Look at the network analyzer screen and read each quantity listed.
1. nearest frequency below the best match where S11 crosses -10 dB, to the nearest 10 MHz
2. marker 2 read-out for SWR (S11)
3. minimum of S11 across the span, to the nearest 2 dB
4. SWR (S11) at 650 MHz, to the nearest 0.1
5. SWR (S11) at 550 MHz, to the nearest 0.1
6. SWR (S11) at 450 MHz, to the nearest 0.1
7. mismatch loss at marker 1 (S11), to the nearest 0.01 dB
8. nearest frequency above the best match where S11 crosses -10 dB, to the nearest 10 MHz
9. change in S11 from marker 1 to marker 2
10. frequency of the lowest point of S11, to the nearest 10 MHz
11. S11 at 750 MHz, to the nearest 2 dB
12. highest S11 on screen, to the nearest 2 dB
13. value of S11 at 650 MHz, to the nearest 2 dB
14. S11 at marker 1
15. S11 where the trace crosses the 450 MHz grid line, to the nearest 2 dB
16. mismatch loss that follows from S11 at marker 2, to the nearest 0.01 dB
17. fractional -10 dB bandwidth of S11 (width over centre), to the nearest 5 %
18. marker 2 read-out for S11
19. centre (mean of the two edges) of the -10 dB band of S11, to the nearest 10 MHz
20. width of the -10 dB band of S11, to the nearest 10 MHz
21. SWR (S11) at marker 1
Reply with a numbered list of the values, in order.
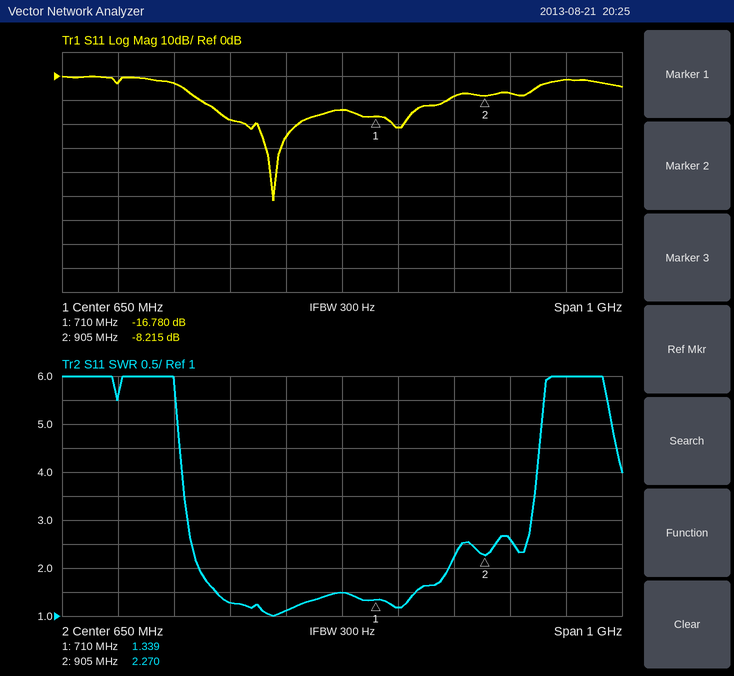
1. 400 MHz
2. 2.270
3. -52 dB
4. 1.5
5. 1.1
6. 1.3
7. 0.09 dB
8. 840 MHz
9. 8.565 dB
10. 530 MHz
11. -22 dB
12. 0 dB
13. -14 dB
14. -16.780 dB
15. -18 dB
16. 0.71 dB
17. 70 %
18. -8.215 dB
19. 620 MHz
20. 440 MHz
21. 1.339
